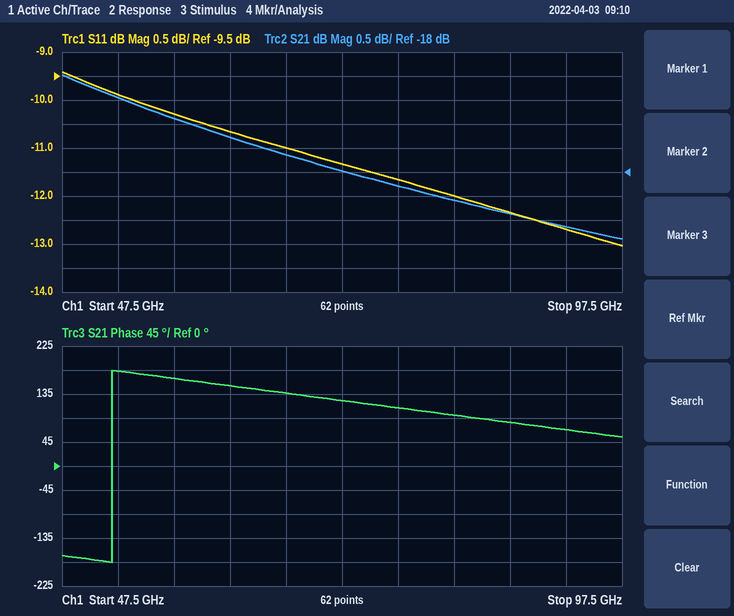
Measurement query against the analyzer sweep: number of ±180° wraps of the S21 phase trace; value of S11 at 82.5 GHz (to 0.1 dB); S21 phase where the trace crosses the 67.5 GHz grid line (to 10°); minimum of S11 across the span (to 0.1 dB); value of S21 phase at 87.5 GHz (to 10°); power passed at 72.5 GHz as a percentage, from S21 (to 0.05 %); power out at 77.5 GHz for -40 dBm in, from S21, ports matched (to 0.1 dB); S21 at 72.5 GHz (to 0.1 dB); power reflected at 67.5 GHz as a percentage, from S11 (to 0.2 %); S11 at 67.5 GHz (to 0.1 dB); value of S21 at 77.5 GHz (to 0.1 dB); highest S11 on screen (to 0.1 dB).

1
-12.0 dB
140°
-13.0 dB
80°
1.60 %
-58.3 dBm
-18.0 dB
8.0 %
-11.0 dB
-18.3 dB
-9.4 dB
